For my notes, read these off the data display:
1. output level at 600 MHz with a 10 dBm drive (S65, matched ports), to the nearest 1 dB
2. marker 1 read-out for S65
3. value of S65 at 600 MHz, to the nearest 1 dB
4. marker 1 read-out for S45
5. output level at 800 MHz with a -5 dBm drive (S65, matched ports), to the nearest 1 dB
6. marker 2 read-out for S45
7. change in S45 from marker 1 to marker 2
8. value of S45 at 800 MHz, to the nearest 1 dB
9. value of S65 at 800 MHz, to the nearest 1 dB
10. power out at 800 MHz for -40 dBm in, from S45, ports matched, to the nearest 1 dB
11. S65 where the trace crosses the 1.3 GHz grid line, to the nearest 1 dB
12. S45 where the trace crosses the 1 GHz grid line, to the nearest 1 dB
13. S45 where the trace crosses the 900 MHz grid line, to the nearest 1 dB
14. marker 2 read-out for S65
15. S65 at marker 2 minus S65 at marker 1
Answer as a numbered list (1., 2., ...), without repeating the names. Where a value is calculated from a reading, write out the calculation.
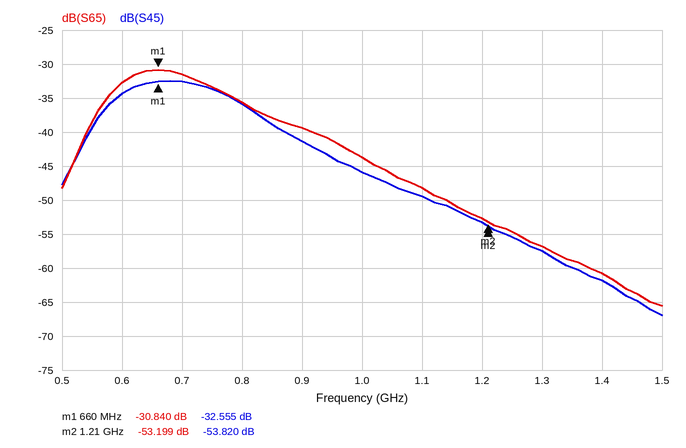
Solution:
1. 10 dBm + (-33 dB) = -23 dBm
2. -30.840 dB
3. -33 dB
4. -32.555 dB
5. -5 dBm + (-36 dB) = -41 dBm
6. -53.820 dB
7. -53.82 − (-32.555) = -21.265 dB
8. -36 dB
9. -36 dB
10. -40 dBm + (-36 dB) = -76 dBm
11. -57 dB
12. -46 dB
13. -41 dB
14. -53.199 dB
15. -53.199 − (-30.84) = -22.359 dB
